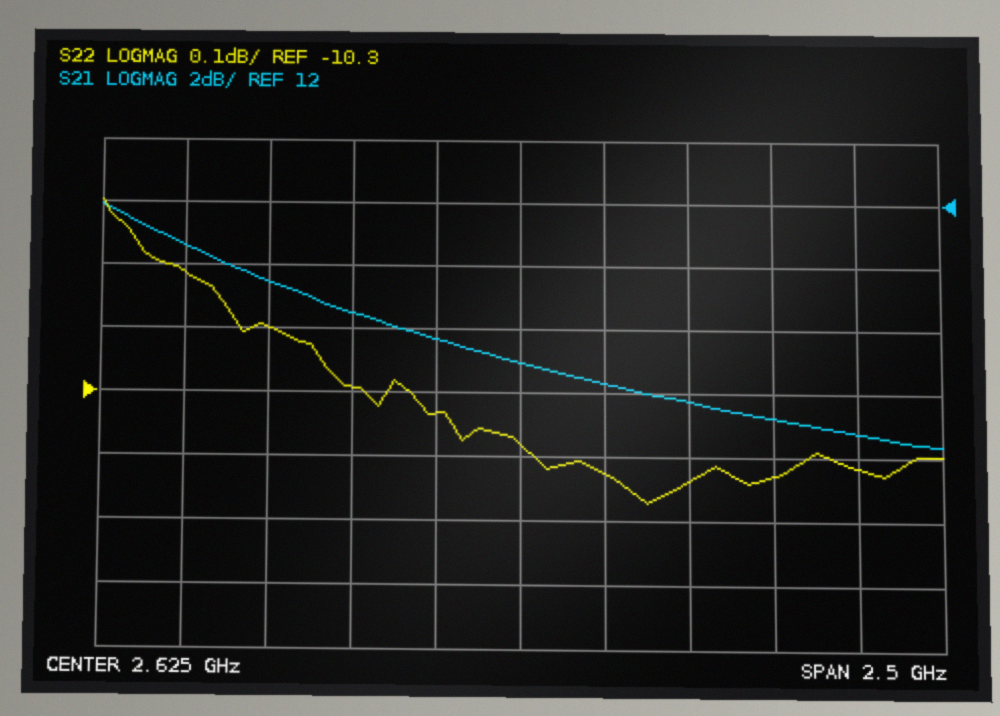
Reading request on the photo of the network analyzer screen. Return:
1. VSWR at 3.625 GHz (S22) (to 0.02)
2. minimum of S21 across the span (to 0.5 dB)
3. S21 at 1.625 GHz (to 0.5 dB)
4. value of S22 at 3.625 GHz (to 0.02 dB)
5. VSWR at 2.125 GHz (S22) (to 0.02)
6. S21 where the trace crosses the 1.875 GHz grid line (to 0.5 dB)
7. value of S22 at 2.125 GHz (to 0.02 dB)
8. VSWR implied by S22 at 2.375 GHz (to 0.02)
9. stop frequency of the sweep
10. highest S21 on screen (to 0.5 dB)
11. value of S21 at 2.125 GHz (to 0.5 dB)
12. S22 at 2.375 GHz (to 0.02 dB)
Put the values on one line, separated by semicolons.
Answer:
1.86; 4.5 dB; 10.5 dB; -10.42 dB; 1.88; 9.5 dB; -10.30 dB; 1.88; 3.875 GHz; 12.0 dB; 8.5 dB; -10.34 dB
